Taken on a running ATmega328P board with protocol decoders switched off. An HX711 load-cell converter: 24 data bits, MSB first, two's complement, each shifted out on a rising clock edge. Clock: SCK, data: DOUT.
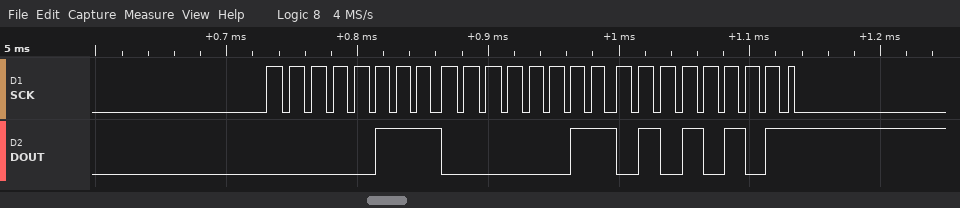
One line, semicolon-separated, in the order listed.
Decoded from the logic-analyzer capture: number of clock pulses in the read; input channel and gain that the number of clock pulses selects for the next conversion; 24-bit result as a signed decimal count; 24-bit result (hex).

25; channel A, gain 128; 459605; 0x070355
